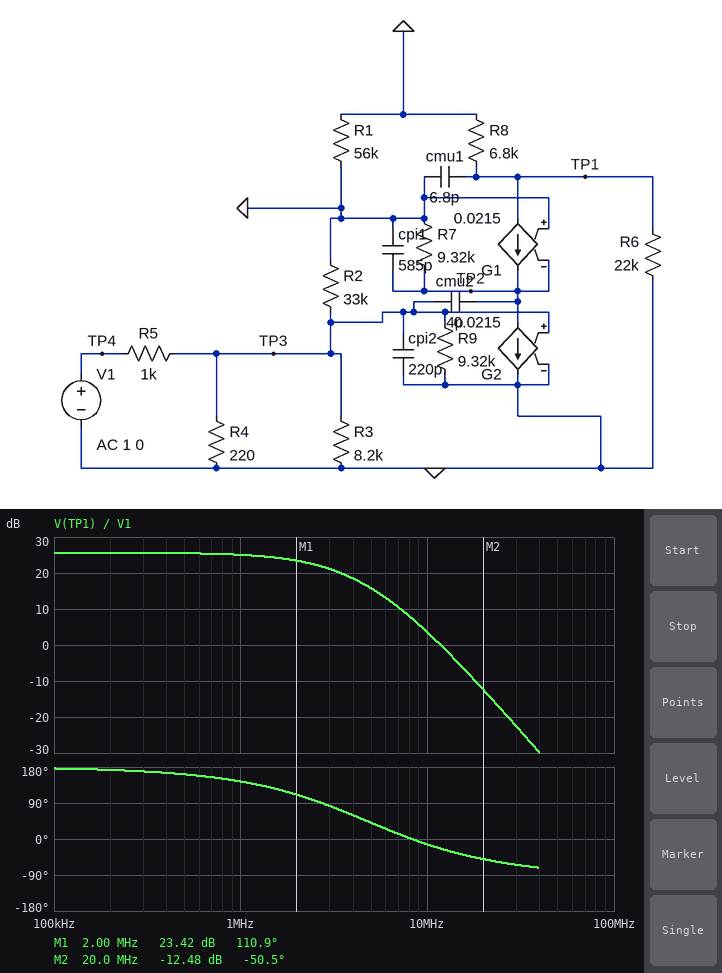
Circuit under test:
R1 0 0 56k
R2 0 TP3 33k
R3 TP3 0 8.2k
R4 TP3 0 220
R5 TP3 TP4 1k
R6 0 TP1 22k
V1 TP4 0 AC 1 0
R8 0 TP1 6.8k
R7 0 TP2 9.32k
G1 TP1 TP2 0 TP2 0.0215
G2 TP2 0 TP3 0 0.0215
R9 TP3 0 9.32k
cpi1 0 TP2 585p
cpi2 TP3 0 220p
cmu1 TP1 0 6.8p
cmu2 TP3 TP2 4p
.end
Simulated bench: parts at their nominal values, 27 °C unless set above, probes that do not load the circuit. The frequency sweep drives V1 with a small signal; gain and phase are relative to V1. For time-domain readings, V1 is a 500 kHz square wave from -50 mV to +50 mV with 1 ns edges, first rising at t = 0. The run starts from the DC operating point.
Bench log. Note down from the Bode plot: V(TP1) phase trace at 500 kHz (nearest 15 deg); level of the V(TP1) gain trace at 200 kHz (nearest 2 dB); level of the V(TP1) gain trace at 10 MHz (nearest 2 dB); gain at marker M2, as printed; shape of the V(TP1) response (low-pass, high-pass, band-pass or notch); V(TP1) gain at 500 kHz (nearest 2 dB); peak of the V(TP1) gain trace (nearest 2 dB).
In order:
165 deg
26 dB
4 dB
-12.48 dB
low-pass
26 dB
26 dB
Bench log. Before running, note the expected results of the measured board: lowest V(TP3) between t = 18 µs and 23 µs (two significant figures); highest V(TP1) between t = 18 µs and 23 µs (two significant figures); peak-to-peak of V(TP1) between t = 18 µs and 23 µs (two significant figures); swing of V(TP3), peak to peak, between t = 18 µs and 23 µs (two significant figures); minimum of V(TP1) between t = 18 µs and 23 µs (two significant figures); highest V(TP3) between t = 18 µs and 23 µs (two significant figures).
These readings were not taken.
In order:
-8.6 mV
960 mV
1.9 V
17 mV
-960 mV
8.6 mV
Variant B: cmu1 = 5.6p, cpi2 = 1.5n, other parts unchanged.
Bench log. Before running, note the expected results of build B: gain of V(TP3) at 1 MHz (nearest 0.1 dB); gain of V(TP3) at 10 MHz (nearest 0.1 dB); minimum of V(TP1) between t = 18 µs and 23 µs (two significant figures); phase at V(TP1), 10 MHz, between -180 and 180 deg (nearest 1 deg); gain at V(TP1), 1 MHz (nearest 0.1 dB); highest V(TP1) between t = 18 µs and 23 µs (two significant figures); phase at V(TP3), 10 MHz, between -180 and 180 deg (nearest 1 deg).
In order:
-20.9 dB
-39.5 dB
-910 mV
-28 deg
19.7 dB
910 mV
-86 deg
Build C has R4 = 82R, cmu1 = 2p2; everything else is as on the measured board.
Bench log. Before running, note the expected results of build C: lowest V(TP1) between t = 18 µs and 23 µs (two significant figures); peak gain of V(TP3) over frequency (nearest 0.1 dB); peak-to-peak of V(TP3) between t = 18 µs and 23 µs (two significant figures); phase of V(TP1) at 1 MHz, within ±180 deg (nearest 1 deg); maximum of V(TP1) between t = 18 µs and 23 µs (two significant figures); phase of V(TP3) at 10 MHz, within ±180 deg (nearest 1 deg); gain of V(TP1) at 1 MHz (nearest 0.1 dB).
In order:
-410 mV
-22.6 dB
7.4 mV
160 deg
410 mV
-46 deg
18.1 dB
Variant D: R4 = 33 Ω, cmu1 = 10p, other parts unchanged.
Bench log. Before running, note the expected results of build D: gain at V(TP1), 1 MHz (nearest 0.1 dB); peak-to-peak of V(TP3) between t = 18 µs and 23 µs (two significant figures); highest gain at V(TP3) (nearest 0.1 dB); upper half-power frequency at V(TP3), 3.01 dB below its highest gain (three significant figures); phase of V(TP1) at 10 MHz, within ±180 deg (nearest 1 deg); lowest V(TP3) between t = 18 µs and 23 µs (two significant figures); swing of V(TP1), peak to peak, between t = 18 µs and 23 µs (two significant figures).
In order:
10.4 dB
3.2 mV
-30.0 dB
22.3 MHz
23 deg
-1.6 mV
350 mV
